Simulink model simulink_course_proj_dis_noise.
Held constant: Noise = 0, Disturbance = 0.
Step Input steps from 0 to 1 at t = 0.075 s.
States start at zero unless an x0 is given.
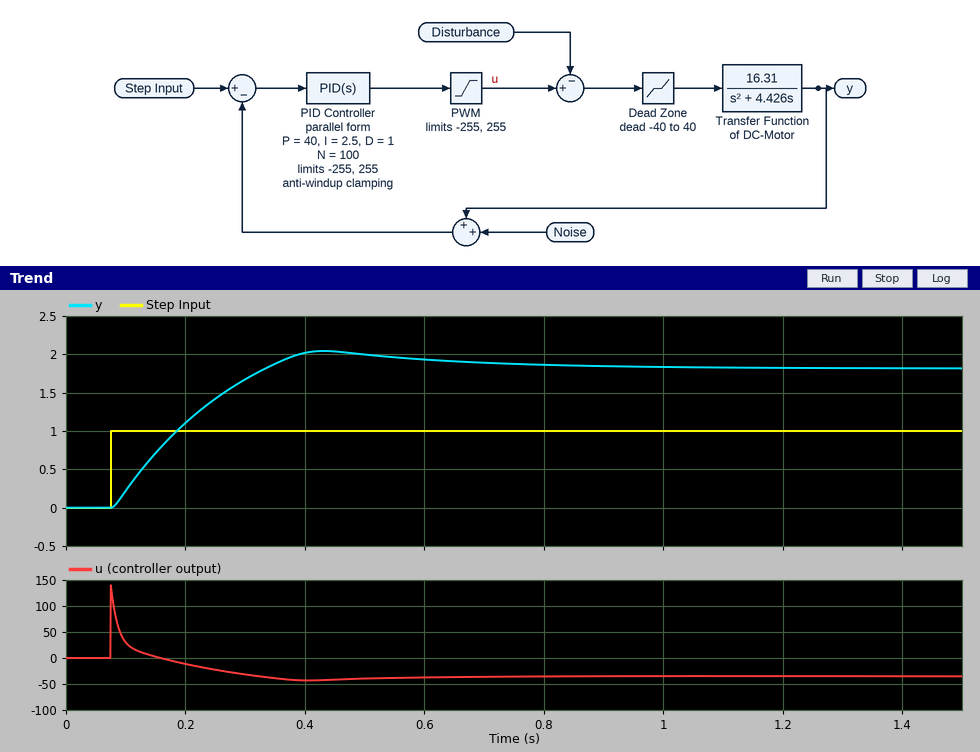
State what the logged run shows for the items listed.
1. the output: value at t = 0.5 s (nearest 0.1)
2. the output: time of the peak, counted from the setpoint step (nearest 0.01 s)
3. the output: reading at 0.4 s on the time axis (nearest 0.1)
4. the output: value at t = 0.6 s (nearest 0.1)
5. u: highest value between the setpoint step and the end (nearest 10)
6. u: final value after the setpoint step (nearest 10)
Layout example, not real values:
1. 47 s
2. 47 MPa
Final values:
1. 2.0
2. 0.36 s
3. 2.0
4. 1.9
5. 140
6. -40
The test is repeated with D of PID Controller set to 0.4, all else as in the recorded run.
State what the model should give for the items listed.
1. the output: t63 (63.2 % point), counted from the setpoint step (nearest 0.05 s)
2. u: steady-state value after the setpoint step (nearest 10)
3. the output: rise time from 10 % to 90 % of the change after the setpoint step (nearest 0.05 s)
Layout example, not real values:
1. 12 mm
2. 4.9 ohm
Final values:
1. 0.25 s
2. -10
3. 0.50 s
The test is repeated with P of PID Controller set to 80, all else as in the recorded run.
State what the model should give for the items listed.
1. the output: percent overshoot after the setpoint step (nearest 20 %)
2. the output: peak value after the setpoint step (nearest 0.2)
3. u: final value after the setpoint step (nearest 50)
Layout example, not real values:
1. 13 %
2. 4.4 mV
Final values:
1. 160 %
2. 1.8
3. 50
